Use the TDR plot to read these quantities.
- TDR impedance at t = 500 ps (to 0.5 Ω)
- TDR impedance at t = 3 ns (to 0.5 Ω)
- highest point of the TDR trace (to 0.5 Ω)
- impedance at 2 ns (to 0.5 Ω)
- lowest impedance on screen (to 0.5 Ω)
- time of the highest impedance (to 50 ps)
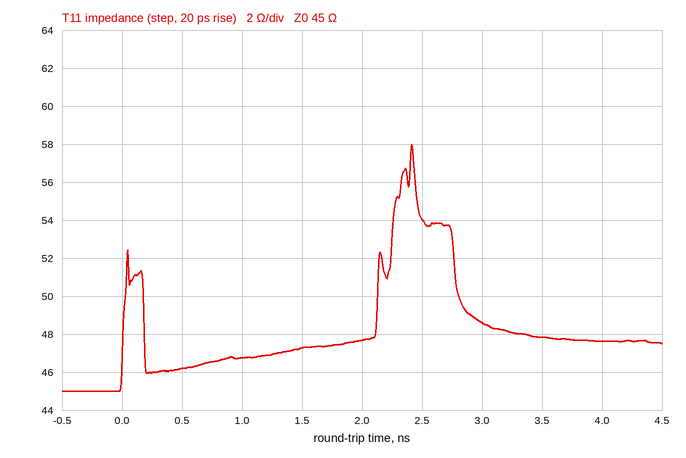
46.0 Ω
48.5 Ω
58.0 Ω
47.5 Ω
45.0 Ω
2.40 ns
